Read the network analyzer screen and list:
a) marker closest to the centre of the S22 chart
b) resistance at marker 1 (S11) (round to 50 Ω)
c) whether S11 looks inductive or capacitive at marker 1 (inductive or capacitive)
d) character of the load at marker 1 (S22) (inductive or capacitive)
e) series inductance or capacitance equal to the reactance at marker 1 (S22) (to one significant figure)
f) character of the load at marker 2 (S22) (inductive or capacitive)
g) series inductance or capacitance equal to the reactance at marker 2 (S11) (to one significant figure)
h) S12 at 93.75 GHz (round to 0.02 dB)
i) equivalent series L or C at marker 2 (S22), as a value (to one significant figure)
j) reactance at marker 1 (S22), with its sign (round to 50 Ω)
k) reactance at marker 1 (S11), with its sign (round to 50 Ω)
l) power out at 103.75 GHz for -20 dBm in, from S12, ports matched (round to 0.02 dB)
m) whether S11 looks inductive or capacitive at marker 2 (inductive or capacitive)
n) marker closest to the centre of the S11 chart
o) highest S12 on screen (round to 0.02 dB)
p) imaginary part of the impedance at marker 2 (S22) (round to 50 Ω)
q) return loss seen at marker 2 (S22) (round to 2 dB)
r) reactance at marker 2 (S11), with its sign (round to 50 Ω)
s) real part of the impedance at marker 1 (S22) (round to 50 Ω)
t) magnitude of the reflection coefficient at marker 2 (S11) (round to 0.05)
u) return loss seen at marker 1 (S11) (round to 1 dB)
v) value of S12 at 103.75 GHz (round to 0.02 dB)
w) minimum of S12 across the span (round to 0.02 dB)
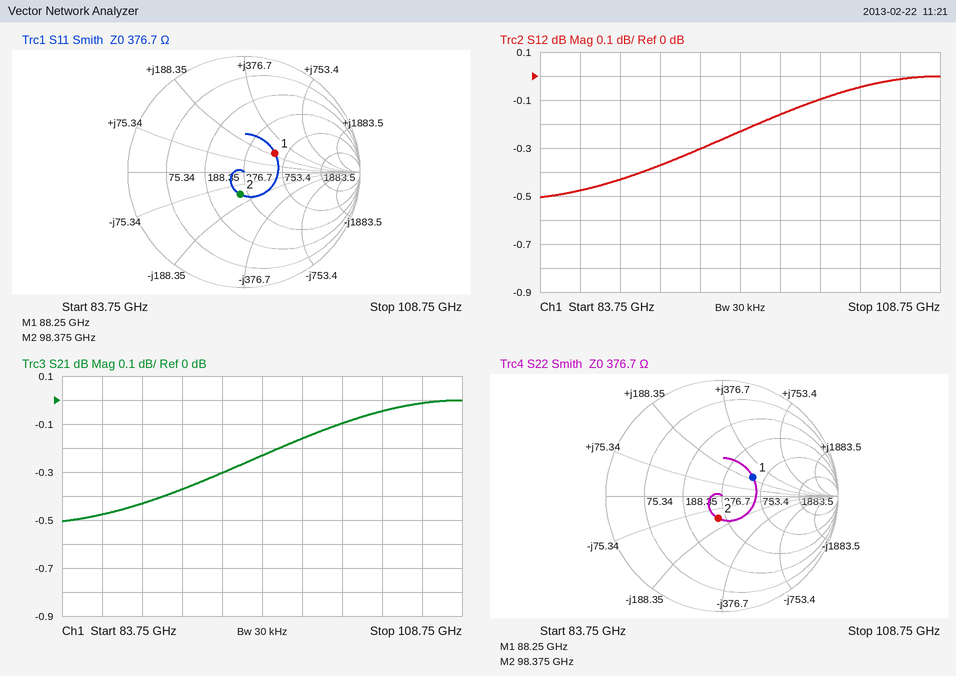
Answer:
marker 2
600 Ω
inductive
inductive
400 pH
capacitive
10 fF
-0.30 dB
10 fF
+200 Ω
+200 Ω
-20.04 dBm
capacitive
marker 2
0.00 dB
-150 Ω
14 dB
-150 Ω
600 Ω
0.20
10 dB
-0.04 dB
-0.50 dB
